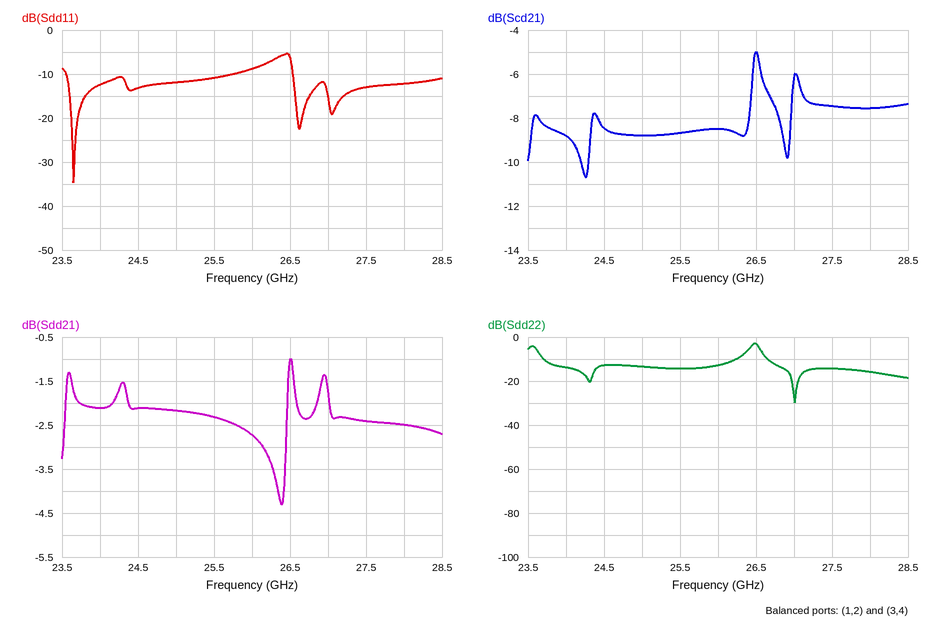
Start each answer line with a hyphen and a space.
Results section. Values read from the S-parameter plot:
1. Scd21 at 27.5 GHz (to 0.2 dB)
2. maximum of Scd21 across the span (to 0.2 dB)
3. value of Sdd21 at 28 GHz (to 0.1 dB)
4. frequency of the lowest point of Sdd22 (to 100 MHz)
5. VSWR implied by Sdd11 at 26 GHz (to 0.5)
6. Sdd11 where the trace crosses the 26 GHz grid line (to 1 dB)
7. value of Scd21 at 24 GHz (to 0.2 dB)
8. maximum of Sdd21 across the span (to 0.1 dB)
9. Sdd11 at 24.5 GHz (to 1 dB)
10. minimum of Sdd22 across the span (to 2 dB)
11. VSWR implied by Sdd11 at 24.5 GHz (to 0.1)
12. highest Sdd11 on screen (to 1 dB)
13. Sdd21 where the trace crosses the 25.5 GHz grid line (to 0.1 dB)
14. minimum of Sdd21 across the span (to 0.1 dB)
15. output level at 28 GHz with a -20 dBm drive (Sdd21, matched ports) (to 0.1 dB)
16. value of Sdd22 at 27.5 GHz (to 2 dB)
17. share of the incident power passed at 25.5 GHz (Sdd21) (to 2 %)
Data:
- -7.4 dB
- -5.0 dB
- -2.5 dB
- 27.0 GHz
- 2.0
- -9 dB
- -8.8 dB
- -1.0 dB
- -13 dB
- -30 dB
- 1.6
- -5 dB
- -2.3 dB
- -4.3 dB
- -22.5 dBm
- -14 dB
- 58 %
